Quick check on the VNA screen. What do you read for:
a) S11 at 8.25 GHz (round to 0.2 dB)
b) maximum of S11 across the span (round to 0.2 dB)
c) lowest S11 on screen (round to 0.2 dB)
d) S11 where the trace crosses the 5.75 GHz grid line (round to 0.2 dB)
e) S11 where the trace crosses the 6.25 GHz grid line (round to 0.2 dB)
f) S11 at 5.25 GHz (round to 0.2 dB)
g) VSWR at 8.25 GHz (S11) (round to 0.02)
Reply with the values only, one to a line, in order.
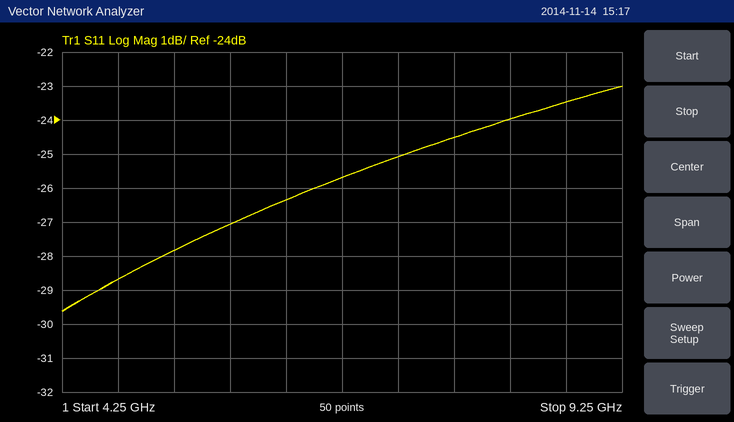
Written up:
-24.0 dB
-23.0 dB
-29.6 dB
-27.0 dB
-26.4 dB
-27.8 dB
1.14
